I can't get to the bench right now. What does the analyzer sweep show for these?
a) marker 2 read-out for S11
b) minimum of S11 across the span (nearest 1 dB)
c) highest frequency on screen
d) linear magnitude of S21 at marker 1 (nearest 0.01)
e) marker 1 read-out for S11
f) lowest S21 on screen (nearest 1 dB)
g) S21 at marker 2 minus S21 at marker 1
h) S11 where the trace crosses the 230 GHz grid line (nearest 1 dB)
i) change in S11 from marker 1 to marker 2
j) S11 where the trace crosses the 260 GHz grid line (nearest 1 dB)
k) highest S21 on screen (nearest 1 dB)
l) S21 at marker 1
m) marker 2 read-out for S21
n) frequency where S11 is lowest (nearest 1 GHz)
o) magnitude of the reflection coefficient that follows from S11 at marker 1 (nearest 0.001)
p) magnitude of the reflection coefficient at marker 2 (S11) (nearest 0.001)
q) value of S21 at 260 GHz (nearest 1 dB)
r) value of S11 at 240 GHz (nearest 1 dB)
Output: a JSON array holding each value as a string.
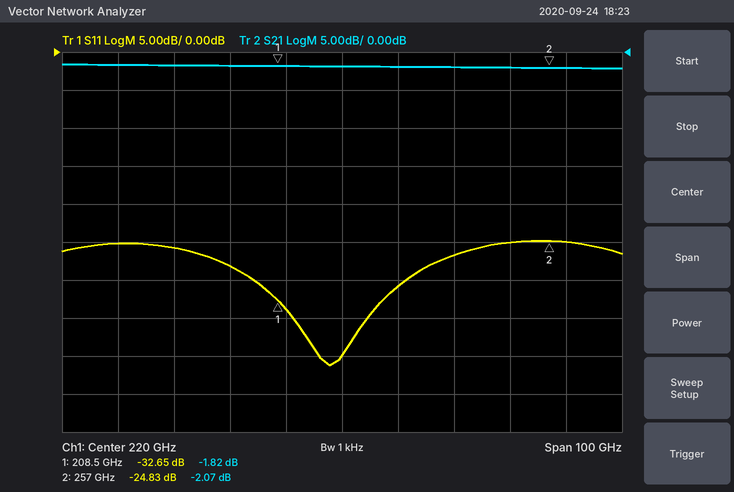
["-24.83 dB", "-41 dB", "270 GHz", "0.81", "-32.65 dB", "-2 dB", "-0.25 dB", "-31 dB", "7.82 dB", "-25 dB", "-2 dB", "-1.82 dB", "-2.07 dB", "218 GHz", "0.023", "0.057", "-2 dB", "-27 dB"]
